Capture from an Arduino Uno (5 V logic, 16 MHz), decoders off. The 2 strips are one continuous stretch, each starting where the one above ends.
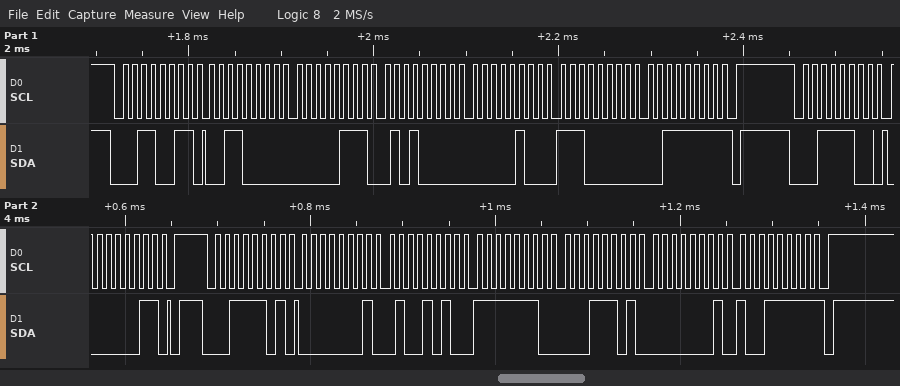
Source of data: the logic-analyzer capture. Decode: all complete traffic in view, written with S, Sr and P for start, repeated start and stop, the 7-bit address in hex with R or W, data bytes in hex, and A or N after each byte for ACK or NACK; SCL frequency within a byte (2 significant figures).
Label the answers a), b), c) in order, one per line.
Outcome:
a) S 19R A 30 A 07 A 50 A 04 A E0 A 3F N P S 1EW A 03 A P S 1ER A 01 A 4A A FE A 1D A 01 A 9F N P
b) 100 kHz
